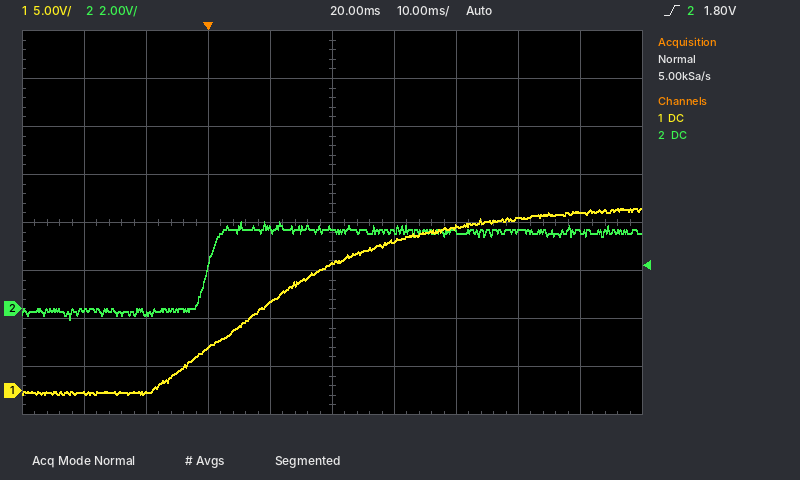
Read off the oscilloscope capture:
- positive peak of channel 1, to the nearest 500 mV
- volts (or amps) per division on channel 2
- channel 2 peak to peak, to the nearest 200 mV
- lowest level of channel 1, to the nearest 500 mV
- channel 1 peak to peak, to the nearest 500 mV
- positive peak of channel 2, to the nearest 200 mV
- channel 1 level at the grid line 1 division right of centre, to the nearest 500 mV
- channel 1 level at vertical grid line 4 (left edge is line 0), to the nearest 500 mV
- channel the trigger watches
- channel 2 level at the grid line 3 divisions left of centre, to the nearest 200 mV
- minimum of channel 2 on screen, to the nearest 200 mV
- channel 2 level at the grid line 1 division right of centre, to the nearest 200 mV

19.0 V
2 V
4.0 V
-500 mV
19.5 V
3.6 V
15.5 V
9.0 V
channel 2
-200 mV
-400 mV
3.2 V
